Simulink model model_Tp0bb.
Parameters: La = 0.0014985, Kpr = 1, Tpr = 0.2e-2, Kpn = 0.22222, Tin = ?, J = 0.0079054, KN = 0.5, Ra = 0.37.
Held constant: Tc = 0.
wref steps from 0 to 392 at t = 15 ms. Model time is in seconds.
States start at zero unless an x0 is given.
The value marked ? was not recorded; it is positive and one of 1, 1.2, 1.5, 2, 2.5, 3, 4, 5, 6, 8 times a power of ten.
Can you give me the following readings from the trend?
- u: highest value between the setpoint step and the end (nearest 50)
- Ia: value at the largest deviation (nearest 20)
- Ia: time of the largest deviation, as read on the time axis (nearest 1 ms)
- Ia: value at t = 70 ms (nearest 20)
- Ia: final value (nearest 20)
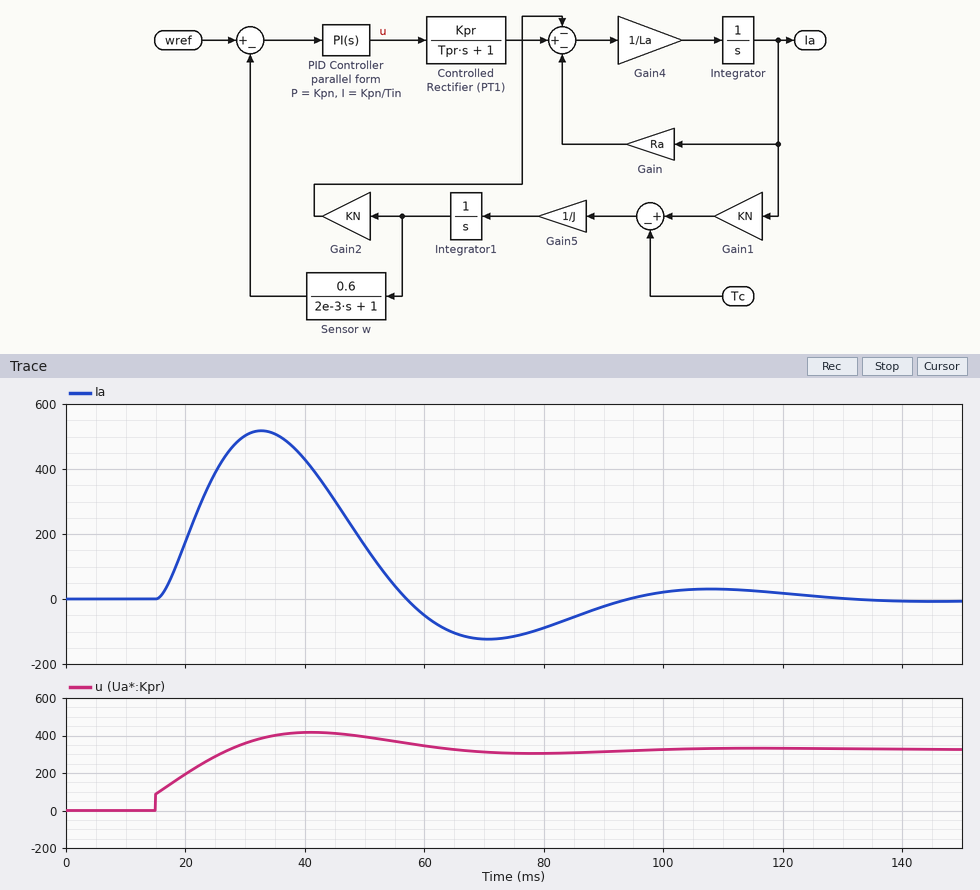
400
520
33 ms
-120
0
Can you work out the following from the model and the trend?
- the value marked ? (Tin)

0.004
